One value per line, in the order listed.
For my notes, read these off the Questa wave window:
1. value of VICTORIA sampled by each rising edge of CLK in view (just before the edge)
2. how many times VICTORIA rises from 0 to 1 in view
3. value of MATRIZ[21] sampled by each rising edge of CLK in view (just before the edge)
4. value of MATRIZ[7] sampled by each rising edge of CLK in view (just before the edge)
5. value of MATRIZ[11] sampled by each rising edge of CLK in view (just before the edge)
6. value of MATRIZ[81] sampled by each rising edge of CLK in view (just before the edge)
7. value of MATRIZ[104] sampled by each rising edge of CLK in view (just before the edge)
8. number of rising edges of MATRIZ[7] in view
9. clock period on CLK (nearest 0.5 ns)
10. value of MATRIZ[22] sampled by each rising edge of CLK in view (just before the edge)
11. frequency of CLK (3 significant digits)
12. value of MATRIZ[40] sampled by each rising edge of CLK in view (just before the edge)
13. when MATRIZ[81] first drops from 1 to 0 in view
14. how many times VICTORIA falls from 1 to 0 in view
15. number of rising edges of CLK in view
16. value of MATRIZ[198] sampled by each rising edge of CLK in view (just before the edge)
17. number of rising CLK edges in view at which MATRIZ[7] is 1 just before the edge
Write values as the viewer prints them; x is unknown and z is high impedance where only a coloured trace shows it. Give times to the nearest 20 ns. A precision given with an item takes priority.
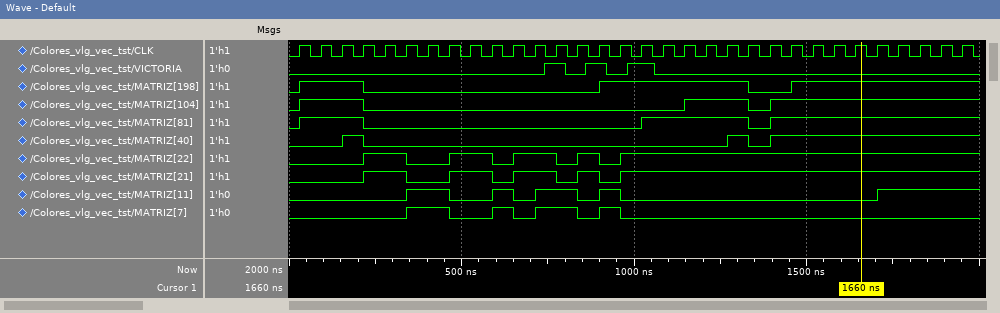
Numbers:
0 0 0 0 0 0 0 0 0 0 0 0 1 0 1 0 1 0 0 0 0 0 0 0 0 0 0 0 0 0 0 0
3
0 0 0 0 1 1 0 0 1 1 0 1 1 0 1 0 1 1 1 1 1 1 1 1 1 1 1 1 1 1 1 1
0 0 0 0 0 0 1 1 0 0 1 0 1 1 0 1 0 0 0 0 0 0 0 0 0 0 0 0 0 0 0 0
0 0 0 0 0 0 1 1 0 0 1 0 1 1 0 1 0 0 0 0 0 0 0 0 0 0 0 0 1 1 1 1
0 1 1 1 0 0 0 0 0 0 0 0 0 0 0 0 0 1 1 1 1 1 0 1 1 1 1 1 1 1 1 1
0 1 1 1 0 0 0 0 0 0 0 0 0 0 0 0 0 0 0 1 1 1 0 1 1 1 1 1 1 1 1 1
4
62 ns
0 0 0 0 1 1 0 0 1 1 0 1 1 0 1 0 1 1 1 1 1 1 1 1 1 1 1 1 1 1 1 1
16.1 MHz
0 0 0 1 0 0 0 0 0 0 0 0 0 0 0 0 0 0 0 0 0 1 0 1 1 1 1 1 1 1 1 1
220 ns
3
32
0 1 1 1 0 0 0 0 0 0 0 0 0 0 0 1 1 1 1 1 1 1 0 0 1 1 1 1 1 1 1 1
6
